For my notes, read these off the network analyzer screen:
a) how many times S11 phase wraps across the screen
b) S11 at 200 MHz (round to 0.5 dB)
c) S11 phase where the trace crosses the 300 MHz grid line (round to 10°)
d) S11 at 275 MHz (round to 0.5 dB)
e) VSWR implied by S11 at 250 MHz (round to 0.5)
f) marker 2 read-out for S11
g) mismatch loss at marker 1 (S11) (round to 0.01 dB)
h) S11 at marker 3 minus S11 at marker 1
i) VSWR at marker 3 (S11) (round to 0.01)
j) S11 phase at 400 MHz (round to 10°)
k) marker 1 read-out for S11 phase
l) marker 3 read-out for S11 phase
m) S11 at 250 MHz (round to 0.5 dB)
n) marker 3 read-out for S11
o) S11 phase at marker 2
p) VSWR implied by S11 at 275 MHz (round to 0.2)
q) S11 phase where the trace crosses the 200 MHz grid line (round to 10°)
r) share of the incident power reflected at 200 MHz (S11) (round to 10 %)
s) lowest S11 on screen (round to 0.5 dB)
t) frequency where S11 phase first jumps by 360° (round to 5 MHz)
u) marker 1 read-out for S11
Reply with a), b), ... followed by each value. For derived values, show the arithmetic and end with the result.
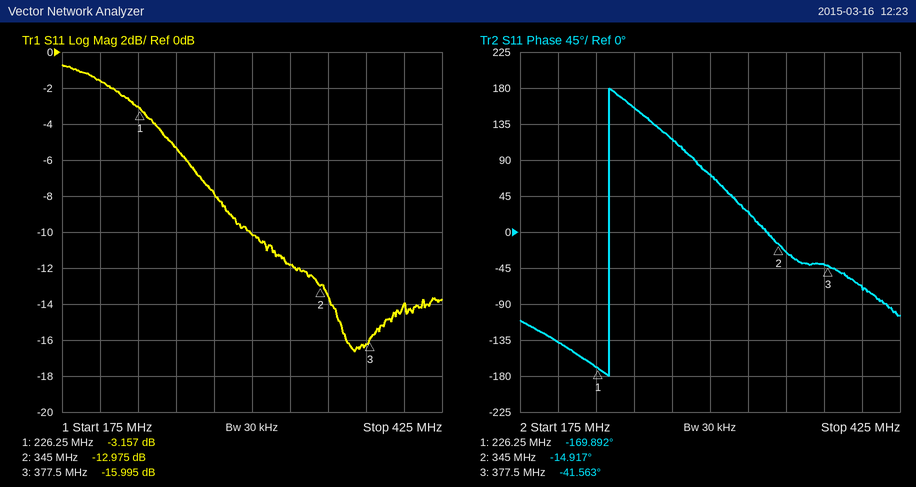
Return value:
a) 1
b) -1.5 dB
c) 70°
d) -8.0 dB
e) |Γ| = 10^(-5.5/20) = 0.5309; VSWR = (1 + 0.5309)/(1 − 0.5309) ≈ 3.26, so 3.5 to the nearest 0.5
f) -12.975 dB
g) −10 log10(1 − 10^(-3.157/10)) ≈ 2.87 dB
h) -15.995 − (-3.157) = -12.838 dB
i) (1 + 0.1586)/(1 − 0.1586) ≈ 1.38
j) -70°
k) -169.892°
l) -41.563°
m) -5.5 dB
n) -15.995 dB
o) -14.917°
p) |Γ| = 10^(-8/20) = 0.3981; VSWR = (1 + 0.3981)/(1 − 0.3981) ≈ 2.32, so 2.4 to the nearest 0.2
q) -140°
r) 10^(-1.5/10) ≈ 70.8 %, so 70 % to the nearest 10 %
s) -16.5 dB
t) 235 MHz
u) -3.157 dB
